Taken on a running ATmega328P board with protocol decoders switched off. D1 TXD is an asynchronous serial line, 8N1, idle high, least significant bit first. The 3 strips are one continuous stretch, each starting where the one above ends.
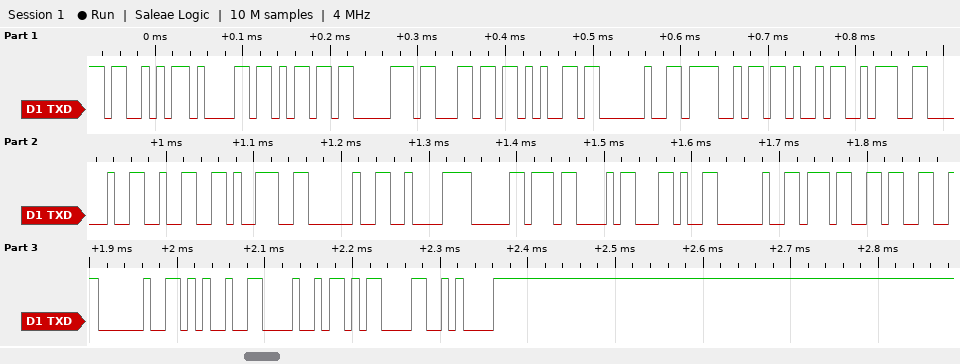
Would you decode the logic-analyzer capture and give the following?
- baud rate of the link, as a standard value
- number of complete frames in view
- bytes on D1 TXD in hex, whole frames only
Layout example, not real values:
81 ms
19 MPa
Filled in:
115200 baud
26
53 61 6D 70 6C 65 20 4F 4B 3A 20 32 39 20 C2 B0 43 2C 20 37 33 20 25 48 0D 0A
